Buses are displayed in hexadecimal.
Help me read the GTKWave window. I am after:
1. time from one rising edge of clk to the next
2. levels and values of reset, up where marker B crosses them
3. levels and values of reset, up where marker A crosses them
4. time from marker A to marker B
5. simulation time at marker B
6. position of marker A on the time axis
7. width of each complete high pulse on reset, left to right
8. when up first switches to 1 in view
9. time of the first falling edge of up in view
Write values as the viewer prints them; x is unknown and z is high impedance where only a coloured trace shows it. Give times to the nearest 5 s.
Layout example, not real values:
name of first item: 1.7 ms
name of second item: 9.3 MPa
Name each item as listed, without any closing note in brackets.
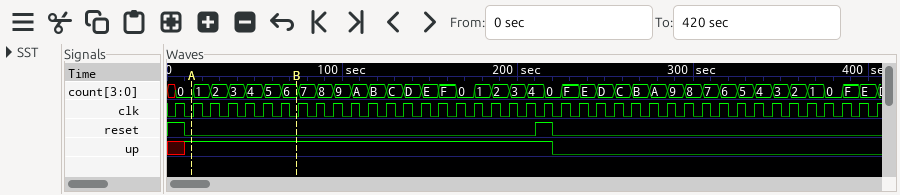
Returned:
time from one rising edge of clk to the next: 10 s
levels and values of reset, up where marker B crosses them: reset=0, up=1
levels and values of reset, up where marker A crosses them: reset=0, up=1
time from marker A to marker B: 60 s
simulation time at marker B: 75 s
position of marker A on the time axis: 15 s
width of each complete high pulse on reset, left to right: 10 s
when up first switches to 1 in view: 10 s
time of the first falling edge of up in view: 220 s
